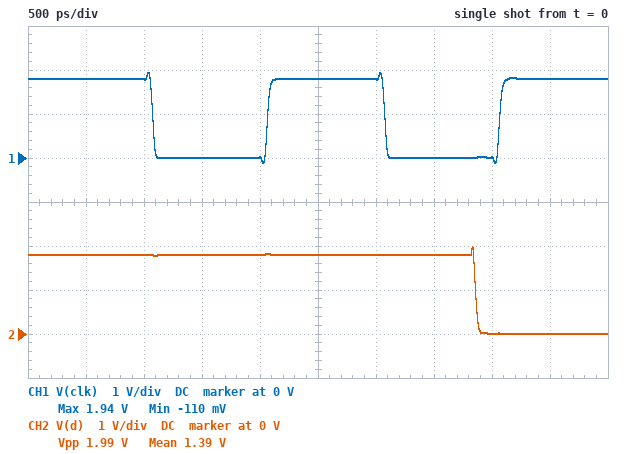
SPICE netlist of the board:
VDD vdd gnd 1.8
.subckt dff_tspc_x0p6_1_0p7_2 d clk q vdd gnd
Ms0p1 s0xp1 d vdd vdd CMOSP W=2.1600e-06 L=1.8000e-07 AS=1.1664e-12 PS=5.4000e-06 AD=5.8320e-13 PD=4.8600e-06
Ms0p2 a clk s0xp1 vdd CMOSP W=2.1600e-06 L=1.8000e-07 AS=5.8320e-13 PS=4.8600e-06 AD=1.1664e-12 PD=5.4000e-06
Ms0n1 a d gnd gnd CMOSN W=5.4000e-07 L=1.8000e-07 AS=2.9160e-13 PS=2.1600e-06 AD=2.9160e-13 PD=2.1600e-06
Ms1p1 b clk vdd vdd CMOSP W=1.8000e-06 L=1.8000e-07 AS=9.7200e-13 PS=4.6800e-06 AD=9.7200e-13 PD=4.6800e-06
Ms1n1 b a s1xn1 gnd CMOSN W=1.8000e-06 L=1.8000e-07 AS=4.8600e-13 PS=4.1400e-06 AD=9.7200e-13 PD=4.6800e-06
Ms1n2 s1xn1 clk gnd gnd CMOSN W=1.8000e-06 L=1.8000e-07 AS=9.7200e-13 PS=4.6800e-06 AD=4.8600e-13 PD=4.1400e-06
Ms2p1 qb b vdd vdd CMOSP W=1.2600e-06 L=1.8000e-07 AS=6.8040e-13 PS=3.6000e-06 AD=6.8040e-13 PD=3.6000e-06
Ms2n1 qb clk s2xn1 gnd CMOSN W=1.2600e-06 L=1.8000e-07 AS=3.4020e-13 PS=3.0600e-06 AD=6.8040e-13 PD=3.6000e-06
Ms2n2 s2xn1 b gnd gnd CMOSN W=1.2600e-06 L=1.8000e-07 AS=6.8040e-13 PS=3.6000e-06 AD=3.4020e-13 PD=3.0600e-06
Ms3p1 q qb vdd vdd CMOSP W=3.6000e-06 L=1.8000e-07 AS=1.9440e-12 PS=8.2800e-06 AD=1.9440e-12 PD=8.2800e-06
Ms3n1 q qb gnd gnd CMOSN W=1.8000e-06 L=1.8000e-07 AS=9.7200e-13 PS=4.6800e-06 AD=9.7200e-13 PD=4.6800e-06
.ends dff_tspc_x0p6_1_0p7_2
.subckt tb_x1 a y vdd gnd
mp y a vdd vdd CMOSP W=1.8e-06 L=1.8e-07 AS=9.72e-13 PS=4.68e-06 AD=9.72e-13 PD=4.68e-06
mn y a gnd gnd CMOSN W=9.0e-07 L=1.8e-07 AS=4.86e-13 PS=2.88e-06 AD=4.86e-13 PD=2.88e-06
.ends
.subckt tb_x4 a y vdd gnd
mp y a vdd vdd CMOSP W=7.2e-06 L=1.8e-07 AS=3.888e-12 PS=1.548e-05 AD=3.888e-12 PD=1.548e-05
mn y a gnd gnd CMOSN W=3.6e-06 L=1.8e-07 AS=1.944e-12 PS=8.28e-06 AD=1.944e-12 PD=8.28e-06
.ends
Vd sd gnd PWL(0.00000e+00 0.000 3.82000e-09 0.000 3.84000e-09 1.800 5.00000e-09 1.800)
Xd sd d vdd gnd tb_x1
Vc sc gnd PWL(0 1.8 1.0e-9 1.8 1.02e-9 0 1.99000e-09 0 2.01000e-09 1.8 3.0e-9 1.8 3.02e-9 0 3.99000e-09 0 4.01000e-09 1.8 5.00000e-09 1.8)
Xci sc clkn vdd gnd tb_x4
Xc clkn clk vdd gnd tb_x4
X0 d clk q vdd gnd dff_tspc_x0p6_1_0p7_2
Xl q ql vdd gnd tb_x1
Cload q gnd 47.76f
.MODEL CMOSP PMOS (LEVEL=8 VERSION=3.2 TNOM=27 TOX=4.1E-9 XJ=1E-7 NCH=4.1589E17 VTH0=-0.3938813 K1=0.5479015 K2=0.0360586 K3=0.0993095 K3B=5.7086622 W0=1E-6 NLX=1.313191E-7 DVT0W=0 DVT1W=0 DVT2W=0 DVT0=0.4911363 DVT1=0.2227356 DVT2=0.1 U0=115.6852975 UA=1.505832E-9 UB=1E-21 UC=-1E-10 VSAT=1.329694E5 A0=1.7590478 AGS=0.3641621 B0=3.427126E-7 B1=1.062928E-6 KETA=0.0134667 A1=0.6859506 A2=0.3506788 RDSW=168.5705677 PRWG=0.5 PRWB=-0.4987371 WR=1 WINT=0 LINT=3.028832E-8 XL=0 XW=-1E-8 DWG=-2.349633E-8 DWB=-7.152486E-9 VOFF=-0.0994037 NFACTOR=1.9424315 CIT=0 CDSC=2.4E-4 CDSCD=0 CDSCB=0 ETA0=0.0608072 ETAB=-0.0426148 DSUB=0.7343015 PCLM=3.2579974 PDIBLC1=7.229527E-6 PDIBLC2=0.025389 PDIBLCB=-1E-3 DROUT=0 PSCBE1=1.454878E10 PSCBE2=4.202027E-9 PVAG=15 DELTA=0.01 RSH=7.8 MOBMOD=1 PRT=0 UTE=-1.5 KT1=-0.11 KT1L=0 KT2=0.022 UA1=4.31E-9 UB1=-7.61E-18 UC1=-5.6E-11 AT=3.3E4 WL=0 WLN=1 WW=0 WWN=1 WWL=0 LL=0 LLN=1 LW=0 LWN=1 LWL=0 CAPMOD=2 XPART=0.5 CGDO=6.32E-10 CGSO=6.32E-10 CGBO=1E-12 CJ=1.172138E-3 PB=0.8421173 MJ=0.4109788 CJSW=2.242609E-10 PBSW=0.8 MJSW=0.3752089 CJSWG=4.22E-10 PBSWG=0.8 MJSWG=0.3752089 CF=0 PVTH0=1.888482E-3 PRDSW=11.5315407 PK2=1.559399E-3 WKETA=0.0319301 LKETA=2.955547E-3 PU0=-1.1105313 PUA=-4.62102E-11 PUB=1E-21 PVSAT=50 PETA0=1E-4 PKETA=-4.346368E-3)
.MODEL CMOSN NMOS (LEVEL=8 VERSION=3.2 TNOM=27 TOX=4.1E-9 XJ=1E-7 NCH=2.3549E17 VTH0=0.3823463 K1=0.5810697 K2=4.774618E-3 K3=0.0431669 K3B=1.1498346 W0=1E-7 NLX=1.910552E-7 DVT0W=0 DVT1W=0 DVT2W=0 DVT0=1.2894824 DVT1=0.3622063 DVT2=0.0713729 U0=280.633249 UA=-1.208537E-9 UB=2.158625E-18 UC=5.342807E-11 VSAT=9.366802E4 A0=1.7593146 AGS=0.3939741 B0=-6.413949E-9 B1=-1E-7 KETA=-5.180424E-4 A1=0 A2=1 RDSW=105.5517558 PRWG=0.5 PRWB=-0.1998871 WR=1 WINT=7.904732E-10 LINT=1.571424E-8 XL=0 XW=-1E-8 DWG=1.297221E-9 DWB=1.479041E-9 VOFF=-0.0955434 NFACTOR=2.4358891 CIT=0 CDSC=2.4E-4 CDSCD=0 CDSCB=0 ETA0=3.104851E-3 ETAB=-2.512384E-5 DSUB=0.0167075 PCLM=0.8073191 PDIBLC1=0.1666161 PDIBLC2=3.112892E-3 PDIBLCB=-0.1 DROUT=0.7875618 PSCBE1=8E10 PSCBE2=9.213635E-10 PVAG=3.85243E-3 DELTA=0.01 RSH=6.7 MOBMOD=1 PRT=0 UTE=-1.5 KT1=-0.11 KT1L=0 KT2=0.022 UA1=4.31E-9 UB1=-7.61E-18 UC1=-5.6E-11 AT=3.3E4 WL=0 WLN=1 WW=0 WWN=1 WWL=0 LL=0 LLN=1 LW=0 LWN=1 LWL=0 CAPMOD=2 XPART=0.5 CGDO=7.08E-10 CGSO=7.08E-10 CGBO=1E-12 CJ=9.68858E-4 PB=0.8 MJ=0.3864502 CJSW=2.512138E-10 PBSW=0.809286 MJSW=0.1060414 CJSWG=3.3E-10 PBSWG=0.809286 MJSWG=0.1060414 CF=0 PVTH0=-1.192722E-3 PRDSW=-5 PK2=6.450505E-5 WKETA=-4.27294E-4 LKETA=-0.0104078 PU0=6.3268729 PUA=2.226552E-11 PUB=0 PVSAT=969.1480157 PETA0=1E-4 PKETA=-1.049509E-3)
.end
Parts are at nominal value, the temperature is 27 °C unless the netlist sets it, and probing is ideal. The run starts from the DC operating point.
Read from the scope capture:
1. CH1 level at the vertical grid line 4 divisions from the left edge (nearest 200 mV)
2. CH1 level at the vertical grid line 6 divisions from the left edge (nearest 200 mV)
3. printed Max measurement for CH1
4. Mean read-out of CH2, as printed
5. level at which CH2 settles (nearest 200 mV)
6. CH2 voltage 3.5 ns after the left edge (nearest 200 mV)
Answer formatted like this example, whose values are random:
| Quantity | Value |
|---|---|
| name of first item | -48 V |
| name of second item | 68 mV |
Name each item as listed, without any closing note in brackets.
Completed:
| Quantity | Value |
|---|---|
| CH1 level at the vertical grid line 4 divisions from the left edge | 0 V |
| CH1 level at the vertical grid line 6 divisions from the left edge | 1.8 V |
| printed Max measurement for CH1 | 1.94 V |
| Mean read-out of CH2, as printed | 1.39 V |
| level at which CH2 settles | 0 V |
| CH2 voltage 3.5 ns after the left edge | 1.8 V |
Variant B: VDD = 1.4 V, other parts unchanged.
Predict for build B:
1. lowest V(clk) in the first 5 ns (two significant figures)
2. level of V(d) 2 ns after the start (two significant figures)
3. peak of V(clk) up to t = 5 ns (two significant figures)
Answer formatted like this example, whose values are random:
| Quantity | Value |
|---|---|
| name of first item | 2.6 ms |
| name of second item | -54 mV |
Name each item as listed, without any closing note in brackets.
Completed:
| Quantity | Value |
|---|---|
| lowest V(clk) in the first 5 ns | -160 mV |
| level of V(d) 2 ns after the start | 1.4 V |
| peak of V(clk) up to t = 5 ns | 1.5 V |
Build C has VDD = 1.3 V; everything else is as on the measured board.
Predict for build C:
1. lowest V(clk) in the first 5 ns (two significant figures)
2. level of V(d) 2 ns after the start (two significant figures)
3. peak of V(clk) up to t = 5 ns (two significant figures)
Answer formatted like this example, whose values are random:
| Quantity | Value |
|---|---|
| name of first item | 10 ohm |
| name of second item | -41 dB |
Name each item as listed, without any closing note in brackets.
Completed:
| Quantity | Value |
|---|---|
| lowest V(clk) in the first 5 ns | -170 mV |
| level of V(d) 2 ns after the start | 1.3 V |
| peak of V(clk) up to t = 5 ns | 1.4 V |
